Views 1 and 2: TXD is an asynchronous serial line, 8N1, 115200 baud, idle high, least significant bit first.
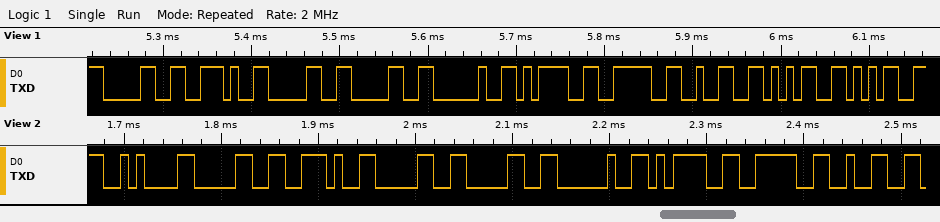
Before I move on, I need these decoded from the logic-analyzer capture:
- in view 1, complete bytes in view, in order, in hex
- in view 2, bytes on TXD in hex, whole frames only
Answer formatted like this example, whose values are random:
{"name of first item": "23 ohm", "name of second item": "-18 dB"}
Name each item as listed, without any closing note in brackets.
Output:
{"in view 1, complete bytes in view, in order, in hex": "30 2E 30 30 20 3D 3E 32 35 35", "in view 2, bytes on TXD in hex, whole frames only": "0A 30 2E 30 30 20 3D 3E 32"}
